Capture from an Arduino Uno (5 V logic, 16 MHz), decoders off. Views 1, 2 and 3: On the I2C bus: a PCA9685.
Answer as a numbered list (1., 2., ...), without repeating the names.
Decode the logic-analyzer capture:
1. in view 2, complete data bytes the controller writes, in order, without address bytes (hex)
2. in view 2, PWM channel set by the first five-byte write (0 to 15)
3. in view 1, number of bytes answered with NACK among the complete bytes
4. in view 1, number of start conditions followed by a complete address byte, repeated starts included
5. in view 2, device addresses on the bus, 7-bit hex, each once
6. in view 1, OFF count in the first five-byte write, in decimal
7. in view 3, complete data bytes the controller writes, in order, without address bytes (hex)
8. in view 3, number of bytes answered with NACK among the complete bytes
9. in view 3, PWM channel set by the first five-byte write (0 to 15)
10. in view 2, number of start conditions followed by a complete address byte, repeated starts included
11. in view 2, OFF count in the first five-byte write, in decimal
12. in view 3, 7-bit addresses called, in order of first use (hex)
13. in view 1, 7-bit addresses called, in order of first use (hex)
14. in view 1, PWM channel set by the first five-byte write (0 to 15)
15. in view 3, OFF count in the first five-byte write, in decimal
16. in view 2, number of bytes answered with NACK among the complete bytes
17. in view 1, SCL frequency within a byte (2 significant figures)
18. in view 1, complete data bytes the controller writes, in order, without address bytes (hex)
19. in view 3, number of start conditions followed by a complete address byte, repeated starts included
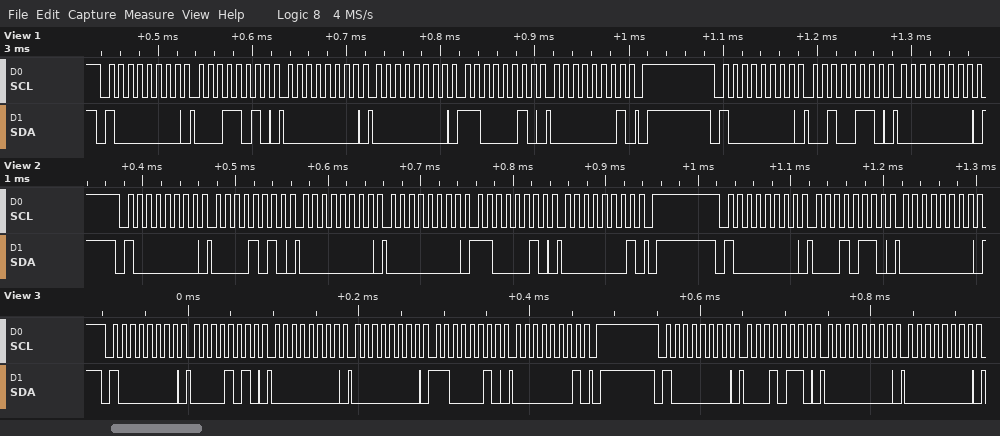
1. 0A 00 00 C2 01 16 00
2. 1
3. 0
4. 2
5. 0x40
6. 450
7. 0A 00 00 C2 01 16 00 00
8. 0
9. 1
10. 2
11. 450
12. 0x40
13. 0x40
14. 5
15. 450
16. 0
17. 100 kHz
18. 1A 00 00 C2 01 26 00
19. 2
